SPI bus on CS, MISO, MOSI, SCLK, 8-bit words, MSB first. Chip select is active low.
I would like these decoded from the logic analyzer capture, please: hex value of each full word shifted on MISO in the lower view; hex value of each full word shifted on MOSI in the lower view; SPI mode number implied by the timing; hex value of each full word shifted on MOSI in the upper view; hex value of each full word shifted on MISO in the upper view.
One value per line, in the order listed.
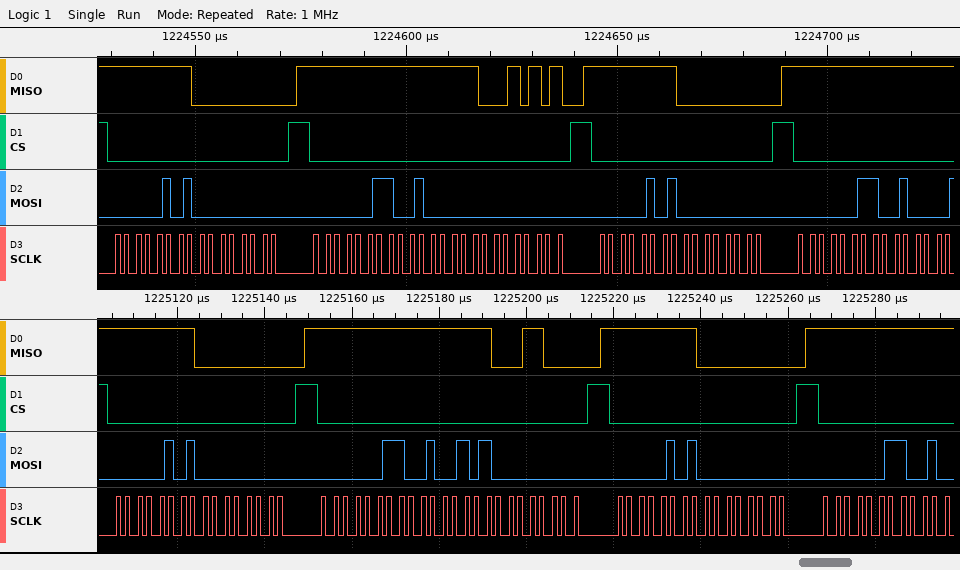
FF, 00, FF, FF, 18, FF, 00, FF
05, 00, 03, 25, 00, 05, 00, 03
0
05, 00, 03, 20, 00, 05, 00, 03
FF, 00, FF, FF, 15, FF, 00, FF
